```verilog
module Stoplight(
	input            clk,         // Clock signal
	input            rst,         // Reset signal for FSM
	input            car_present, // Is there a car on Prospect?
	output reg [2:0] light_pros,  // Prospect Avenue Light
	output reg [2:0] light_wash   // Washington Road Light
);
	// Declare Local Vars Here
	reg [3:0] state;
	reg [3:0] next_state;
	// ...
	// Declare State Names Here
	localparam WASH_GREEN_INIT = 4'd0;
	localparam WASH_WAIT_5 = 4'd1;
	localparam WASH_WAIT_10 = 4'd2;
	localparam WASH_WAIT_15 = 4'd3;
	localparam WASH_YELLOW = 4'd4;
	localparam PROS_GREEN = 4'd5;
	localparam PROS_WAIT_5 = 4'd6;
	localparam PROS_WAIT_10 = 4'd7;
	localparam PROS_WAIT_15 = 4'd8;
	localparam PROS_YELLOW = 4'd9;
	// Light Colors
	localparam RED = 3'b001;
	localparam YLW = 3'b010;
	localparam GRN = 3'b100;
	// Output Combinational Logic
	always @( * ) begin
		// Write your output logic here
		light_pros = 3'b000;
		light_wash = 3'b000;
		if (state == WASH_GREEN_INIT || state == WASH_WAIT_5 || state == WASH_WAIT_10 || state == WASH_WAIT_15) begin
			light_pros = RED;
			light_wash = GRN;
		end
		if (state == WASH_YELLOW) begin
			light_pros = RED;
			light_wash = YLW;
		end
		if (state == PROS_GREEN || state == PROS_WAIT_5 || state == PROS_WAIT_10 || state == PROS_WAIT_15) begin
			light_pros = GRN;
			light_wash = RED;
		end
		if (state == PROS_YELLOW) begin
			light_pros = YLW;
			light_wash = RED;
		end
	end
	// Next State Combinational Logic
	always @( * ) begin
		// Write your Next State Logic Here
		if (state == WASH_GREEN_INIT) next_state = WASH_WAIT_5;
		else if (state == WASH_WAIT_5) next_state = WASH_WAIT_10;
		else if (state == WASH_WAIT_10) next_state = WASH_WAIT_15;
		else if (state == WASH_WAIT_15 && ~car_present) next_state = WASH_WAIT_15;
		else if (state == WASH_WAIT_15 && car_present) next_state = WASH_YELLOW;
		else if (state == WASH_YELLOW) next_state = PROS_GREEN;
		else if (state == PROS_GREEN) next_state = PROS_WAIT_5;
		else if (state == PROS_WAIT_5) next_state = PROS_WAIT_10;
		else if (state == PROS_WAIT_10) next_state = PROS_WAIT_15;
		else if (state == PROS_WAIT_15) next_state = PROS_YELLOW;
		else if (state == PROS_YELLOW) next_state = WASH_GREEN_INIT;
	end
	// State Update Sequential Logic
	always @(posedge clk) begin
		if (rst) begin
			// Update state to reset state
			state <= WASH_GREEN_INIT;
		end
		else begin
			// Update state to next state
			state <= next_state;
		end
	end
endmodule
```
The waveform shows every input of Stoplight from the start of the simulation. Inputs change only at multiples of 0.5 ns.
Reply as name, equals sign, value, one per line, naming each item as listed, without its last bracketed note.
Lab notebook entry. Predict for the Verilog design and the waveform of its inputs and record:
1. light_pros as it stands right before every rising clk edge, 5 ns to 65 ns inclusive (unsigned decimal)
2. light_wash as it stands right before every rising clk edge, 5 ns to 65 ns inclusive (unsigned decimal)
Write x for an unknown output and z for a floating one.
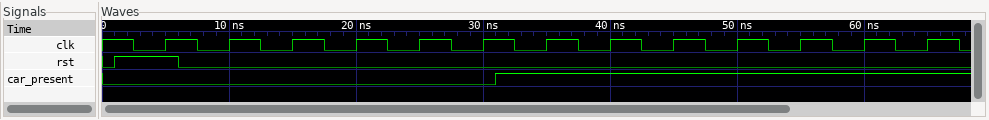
light_pros as it stands right before every rising clk edge, 5 ns to 65 ns inclusive = x, 1, 1, 1, 1, 1, 1, 1, 4, 4, 4, 4, 2
light_wash as it stands right before every rising clk edge, 5 ns to 65 ns inclusive = x, 4, 4, 4, 4, 4, 4, 2, 1, 1, 1, 1, 1
